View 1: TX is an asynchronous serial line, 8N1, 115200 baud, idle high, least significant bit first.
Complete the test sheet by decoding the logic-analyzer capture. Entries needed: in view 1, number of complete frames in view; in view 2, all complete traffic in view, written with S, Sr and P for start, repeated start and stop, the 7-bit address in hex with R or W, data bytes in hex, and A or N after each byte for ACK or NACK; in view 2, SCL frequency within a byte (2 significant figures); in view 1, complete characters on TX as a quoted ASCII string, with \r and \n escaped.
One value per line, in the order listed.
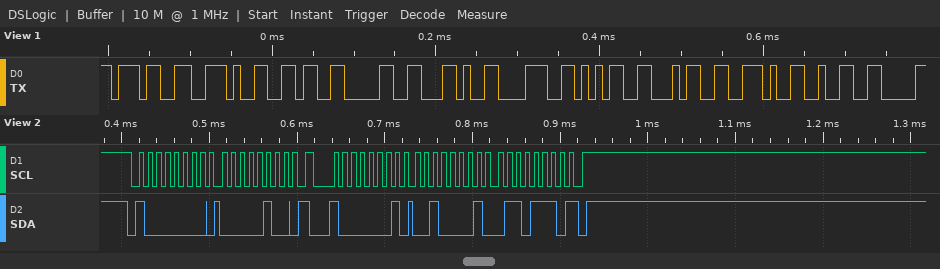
10
S 40W A 04 A Sr 40R A 21 A 6E N P
100 kHz
"7.60,854.2"
